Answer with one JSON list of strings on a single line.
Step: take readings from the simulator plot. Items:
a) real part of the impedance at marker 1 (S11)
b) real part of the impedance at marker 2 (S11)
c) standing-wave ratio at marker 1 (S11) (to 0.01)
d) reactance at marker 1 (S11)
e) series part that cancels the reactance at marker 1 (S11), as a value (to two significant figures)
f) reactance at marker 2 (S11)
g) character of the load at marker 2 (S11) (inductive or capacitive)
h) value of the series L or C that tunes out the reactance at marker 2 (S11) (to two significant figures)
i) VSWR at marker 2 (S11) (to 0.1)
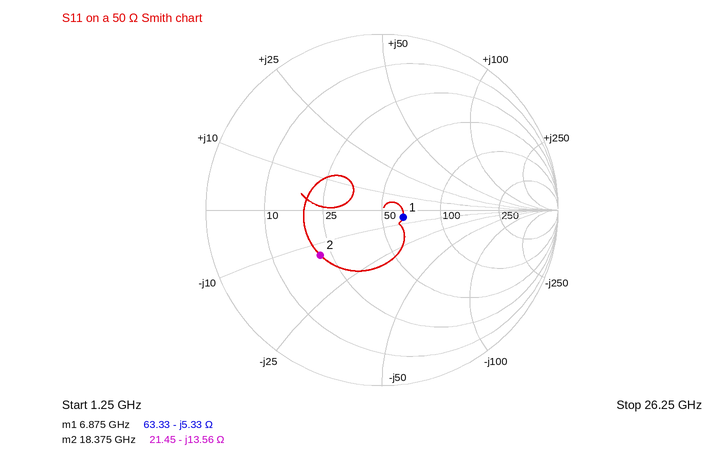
["63.33 Ω", "21.45 Ω", "1.29", "-5.33 Ω", "120 pH", "-13.56 Ω", "capacitive", "120 pH", "2.5"]
